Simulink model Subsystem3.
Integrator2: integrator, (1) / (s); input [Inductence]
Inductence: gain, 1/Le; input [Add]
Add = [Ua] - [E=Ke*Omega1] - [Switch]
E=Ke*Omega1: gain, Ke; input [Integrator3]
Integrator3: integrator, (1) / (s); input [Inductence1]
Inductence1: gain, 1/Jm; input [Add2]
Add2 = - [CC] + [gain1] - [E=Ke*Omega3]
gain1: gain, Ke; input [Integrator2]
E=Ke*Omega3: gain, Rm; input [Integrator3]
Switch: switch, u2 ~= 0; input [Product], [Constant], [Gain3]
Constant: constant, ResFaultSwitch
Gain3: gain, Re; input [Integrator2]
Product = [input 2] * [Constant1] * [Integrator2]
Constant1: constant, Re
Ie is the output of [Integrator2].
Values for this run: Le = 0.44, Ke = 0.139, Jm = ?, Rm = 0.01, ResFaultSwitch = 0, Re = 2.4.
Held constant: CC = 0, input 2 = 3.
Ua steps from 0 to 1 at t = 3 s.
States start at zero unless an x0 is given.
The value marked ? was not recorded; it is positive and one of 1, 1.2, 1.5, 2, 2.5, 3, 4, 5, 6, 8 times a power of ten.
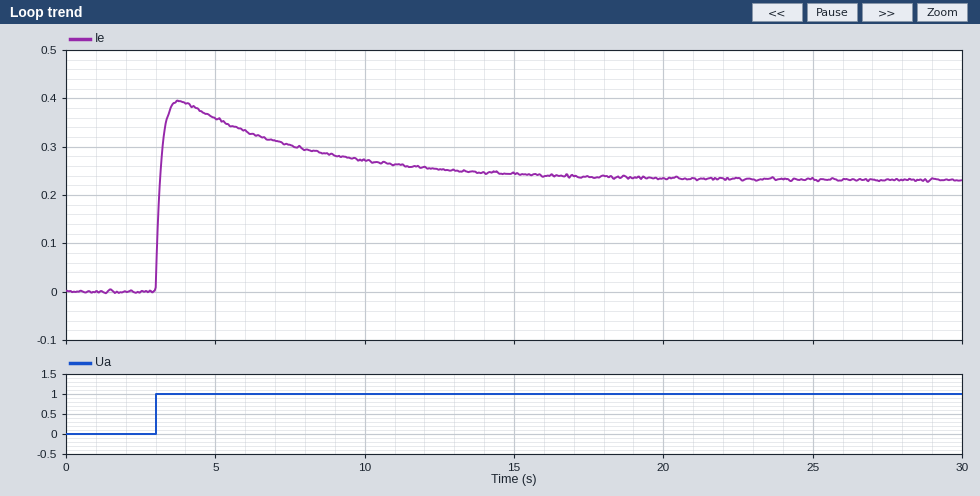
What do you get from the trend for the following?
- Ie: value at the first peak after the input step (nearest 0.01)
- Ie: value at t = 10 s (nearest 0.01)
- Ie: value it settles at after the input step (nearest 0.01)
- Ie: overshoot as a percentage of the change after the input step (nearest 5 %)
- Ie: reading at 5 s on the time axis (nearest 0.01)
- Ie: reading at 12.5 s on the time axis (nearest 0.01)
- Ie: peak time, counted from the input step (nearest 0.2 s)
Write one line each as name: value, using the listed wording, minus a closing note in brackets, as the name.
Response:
Ie: value at the first peak after the input step: 0.39
Ie: value at t = 10 s: 0.27
Ie: value it settles at after the input step: 0.23
Ie: overshoot as a percentage of the change after the input step: 70 %
Ie: reading at 5 s on the time axis: 0.36
Ie: reading at 12.5 s on the time axis: 0.25
Ie: peak time, counted from the input step: 0.8 s
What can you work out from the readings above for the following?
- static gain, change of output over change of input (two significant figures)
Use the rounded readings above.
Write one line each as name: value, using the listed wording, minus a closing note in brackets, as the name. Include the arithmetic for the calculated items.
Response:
static gain, change of output over change of input: (0.23 - 0) / (1 - 0) = 0.23
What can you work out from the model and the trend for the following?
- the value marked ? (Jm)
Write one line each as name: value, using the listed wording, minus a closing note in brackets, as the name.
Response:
the value marked ?: 0.08
